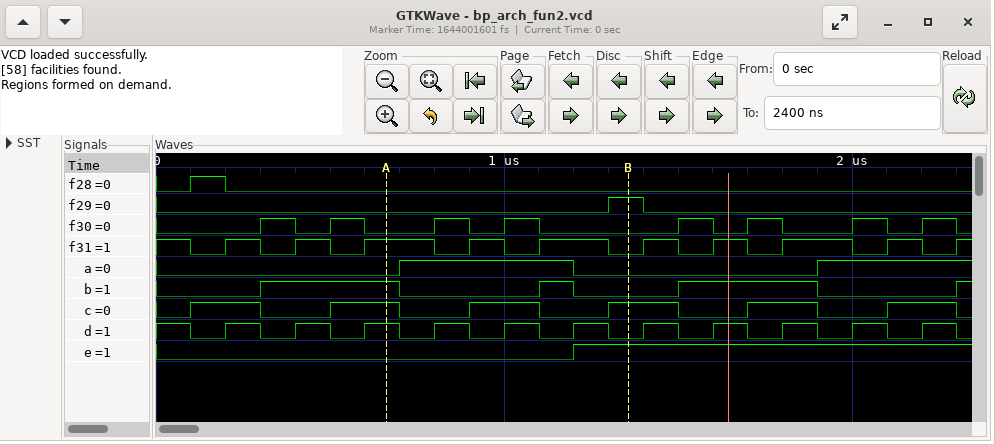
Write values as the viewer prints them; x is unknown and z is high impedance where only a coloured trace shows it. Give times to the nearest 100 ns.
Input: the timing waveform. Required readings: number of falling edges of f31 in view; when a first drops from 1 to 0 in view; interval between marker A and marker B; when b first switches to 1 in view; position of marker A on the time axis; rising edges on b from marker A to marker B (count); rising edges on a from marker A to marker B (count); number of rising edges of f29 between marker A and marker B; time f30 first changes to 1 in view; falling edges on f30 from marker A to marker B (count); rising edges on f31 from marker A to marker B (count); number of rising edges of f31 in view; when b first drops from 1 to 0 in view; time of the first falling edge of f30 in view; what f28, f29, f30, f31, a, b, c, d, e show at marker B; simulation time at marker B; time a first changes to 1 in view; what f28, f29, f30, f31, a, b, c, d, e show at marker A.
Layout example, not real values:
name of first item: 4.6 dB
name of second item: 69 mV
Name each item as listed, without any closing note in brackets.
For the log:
number of falling edges of f31 in view: 10
when a first drops from 1 to 0 in view: 1200 ns
interval between marker A and marker B: 700 ns
when b first switches to 1 in view: 300 ns
position of marker A on the time axis: 700 ns
rising edges on b from marker A to marker B: 1
rising edges on a from marker A to marker B: 1
number of rising edges of f29 between marker A and marker B: 1
time f30 first changes to 1 in view: 300 ns
falling edges on f30 from marker A to marker B: 2
rising edges on f31 from marker A to marker B: 2
number of rising edges of f31 in view: 10
when b first drops from 1 to 0 in view: 700 ns
time of the first falling edge of f30 in view: 400 ns
what f28, f29, f30, f31, a, b, c, d, e show at marker B: f28=0, f29=1, f30=0, f31=0, a=0, b=0, c=1, d=0, e=1
simulation time at marker B: 1400 ns
time a first changes to 1 in view: 700 ns
what f28, f29, f30, f31, a, b, c, d, e show at marker A: f28=0, f29=0, f30=0, f31=1, a=0, b=1, c=1, d=1, e=0
